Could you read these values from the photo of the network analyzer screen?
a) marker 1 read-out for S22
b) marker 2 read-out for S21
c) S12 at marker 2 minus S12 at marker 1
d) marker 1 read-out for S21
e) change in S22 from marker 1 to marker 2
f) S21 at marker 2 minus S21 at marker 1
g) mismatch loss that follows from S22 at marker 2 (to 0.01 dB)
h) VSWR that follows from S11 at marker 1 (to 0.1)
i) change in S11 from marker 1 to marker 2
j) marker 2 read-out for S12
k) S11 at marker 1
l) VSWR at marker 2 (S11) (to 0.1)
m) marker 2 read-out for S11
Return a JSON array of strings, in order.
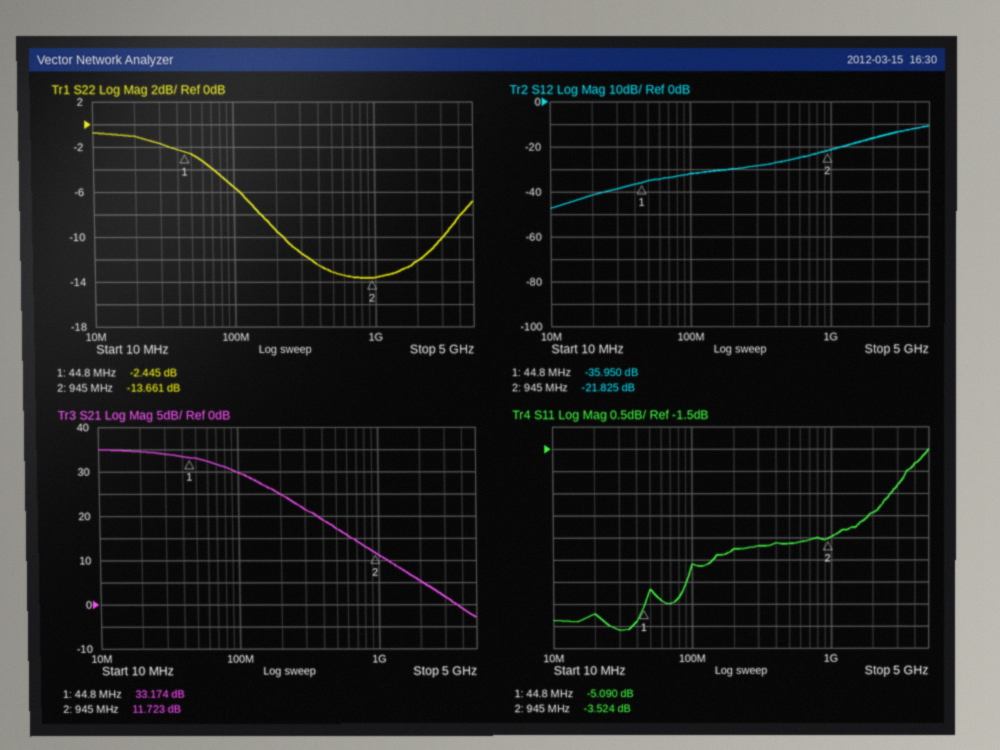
["-2.445 dB", "11.723 dB", "14.125 dB", "33.174 dB", "-11.216 dB", "-21.451 dB", "0.19 dB", "3.5", "1.566 dB", "-21.825 dB", "-5.090 dB", "5.0", "-3.524 dB"]
